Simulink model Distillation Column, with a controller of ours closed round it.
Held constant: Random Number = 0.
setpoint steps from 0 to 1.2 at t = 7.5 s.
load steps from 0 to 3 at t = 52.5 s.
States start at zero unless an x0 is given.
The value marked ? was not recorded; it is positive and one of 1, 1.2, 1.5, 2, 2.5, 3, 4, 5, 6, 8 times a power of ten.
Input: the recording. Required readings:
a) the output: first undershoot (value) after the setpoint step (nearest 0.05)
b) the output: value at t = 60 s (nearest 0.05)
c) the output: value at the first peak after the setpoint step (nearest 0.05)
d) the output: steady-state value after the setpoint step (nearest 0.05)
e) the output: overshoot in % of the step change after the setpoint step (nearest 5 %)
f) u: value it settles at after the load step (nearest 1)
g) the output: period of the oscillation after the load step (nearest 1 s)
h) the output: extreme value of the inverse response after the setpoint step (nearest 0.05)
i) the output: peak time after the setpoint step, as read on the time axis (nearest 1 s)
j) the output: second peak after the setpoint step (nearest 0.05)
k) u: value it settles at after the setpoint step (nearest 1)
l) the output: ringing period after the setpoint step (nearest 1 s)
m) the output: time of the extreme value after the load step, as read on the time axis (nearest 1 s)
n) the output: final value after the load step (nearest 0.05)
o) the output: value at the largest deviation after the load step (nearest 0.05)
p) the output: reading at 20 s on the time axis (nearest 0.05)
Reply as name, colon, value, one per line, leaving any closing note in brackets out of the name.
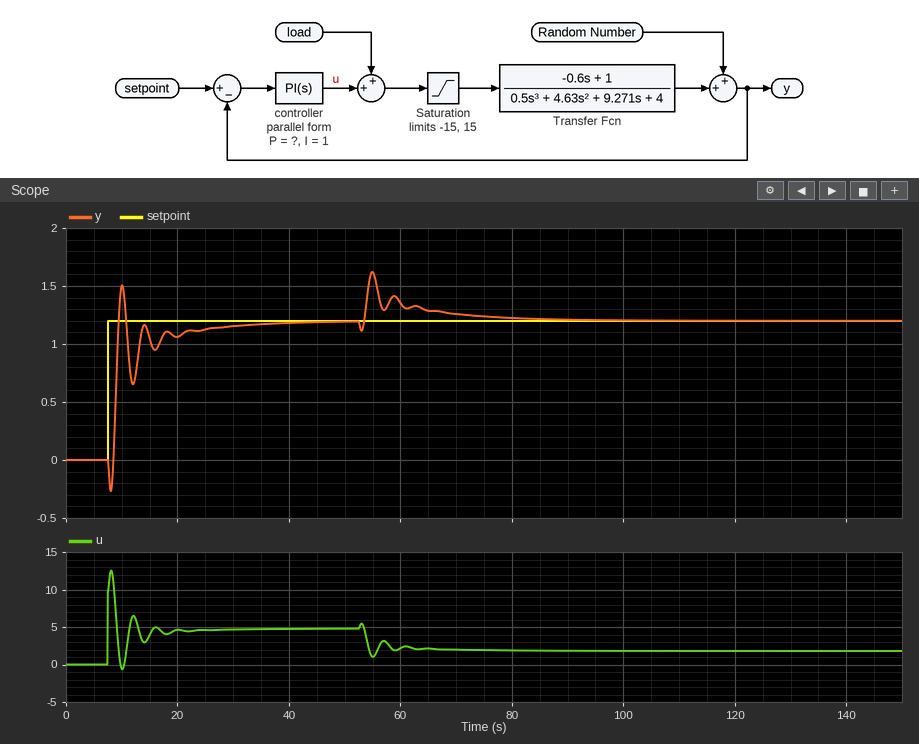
the output: first undershoot (value) after the setpoint step: 0.65
the output: value at t = 60 s: 1.35
the output: value at the first peak after the setpoint step: 1.50
the output: steady-state value after the setpoint step: 1.20
the output: overshoot in % of the step change after the setpoint step: 25 %
u: value it settles at after the load step: 2
the output: period of the oscillation after the load step: 4 s
the output: extreme value of the inverse response after the setpoint step: -0.25
the output: peak time after the setpoint step, as read on the time axis: 10 s
the output: second peak after the setpoint step: 1.15
u: value it settles at after the setpoint step: 5
the output: ringing period after the setpoint step: 4 s
the output: time of the extreme value after the load step, as read on the time axis: 55 s
the output: final value after the load step: 1.20
the output: value at the largest deviation after the load step: 1.60
the output: reading at 20 s on the time axis: 1.05
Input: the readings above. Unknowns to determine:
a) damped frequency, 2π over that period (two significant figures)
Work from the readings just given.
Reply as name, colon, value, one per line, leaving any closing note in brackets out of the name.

damped frequency, 2π over that period: 1.6 rad/s
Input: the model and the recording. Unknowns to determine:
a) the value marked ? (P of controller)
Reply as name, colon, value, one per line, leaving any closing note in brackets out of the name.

the value marked ?: 8
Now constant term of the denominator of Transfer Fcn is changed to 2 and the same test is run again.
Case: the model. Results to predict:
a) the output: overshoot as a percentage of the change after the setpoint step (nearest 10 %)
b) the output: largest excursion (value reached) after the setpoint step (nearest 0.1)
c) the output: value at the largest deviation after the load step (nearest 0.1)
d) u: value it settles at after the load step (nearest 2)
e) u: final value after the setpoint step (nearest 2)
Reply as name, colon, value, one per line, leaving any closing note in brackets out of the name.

the output: overshoot as a percentage of the change after the setpoint step: 40 %
the output: largest excursion (value reached) after the setpoint step: 1.7
the output: value at the largest deviation after the load step: 1.7
u: value it settles at after the load step: 0
u: final value after the setpoint step: 2
